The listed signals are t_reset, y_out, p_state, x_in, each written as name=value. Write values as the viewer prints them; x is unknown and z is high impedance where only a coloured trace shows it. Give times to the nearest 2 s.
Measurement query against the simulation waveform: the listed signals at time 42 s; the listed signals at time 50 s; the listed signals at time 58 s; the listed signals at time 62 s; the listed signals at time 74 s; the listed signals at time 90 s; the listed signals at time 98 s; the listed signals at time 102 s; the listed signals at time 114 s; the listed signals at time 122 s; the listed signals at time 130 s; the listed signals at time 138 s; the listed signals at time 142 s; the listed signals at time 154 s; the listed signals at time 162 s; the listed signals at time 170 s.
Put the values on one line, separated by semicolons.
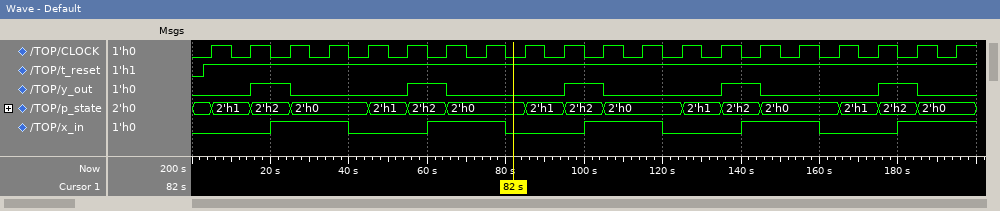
t_reset=1, y_out=0, p_state=2'h0, x_in=0; t_reset=1, y_out=0, p_state=2'h1, x_in=0; t_reset=1, y_out=1, p_state=2'h2, x_in=0; t_reset=1, y_out=1, p_state=2'h2, x_in=1; t_reset=1, y_out=0, p_state=2'h0, x_in=1; t_reset=1, y_out=0, p_state=2'h1, x_in=0; t_reset=1, y_out=1, p_state=2'h2, x_in=0; t_reset=1, y_out=1, p_state=2'h2, x_in=1; t_reset=1, y_out=0, p_state=2'h0, x_in=1; t_reset=1, y_out=0, p_state=2'h0, x_in=0; t_reset=1, y_out=0, p_state=2'h1, x_in=0; t_reset=1, y_out=1, p_state=2'h2, x_in=0; t_reset=1, y_out=1, p_state=2'h2, x_in=1; t_reset=1, y_out=0, p_state=2'h0, x_in=1; t_reset=1, y_out=0, p_state=2'h0, x_in=0; t_reset=1, y_out=0, p_state=2'h1, x_in=0
